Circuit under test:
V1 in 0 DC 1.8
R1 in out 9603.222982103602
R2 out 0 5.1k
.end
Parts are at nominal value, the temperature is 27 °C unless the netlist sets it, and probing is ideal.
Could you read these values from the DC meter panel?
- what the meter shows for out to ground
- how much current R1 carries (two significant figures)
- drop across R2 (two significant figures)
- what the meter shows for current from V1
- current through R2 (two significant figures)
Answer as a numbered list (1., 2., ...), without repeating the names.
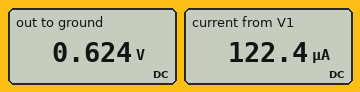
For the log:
1. 0.624 V
2. 120 µA
3. 620 mV
4. 122.4 µA
5. 120 µA
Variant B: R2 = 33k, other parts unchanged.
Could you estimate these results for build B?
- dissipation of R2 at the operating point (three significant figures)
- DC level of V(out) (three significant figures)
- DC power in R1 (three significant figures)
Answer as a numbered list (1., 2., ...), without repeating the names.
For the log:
1. 58.9 µW
2. 1.39 V
3. 17.1 µW
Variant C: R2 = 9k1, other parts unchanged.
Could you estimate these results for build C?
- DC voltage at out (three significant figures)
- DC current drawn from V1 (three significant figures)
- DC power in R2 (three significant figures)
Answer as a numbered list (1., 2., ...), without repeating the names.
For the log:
1. 876 mV
2. 96.2 µA
3. 84.3 µW
